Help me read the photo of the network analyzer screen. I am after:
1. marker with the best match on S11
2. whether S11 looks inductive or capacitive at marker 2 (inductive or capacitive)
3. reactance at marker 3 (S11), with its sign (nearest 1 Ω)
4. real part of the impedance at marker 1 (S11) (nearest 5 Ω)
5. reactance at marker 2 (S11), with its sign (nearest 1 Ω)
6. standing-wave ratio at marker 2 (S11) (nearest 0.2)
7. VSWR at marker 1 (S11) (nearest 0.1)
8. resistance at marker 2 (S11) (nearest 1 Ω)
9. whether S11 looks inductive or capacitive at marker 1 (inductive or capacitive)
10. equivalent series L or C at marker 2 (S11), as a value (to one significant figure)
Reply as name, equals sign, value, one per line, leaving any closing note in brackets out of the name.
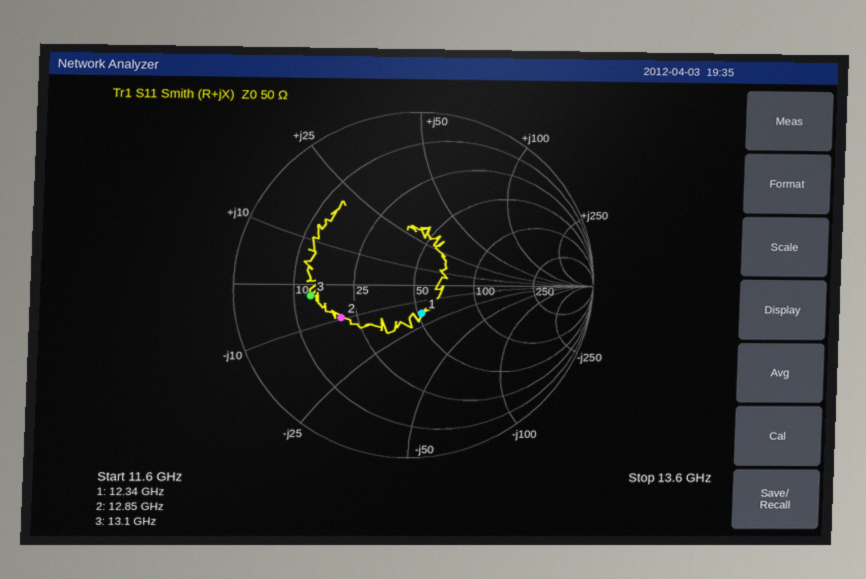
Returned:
marker with the best match on S11 = marker 1
whether S11 looks inductive or capacitive at marker 2 = capacitive
reactance at marker 3 (S11), with its sign = -3 Ω
real part of the impedance at marker 1 (S11) = 50 Ω
reactance at marker 2 (S11), with its sign = -10 Ω
standing-wave ratio at marker 2 (S11) = 2.6
VSWR at marker 1 (S11) = 1.4
resistance at marker 2 (S11) = 20 Ω
whether S11 looks inductive or capacitive at marker 1 = capacitive
equivalent series L or C at marker 2 (S11), as a value = 1 pF
